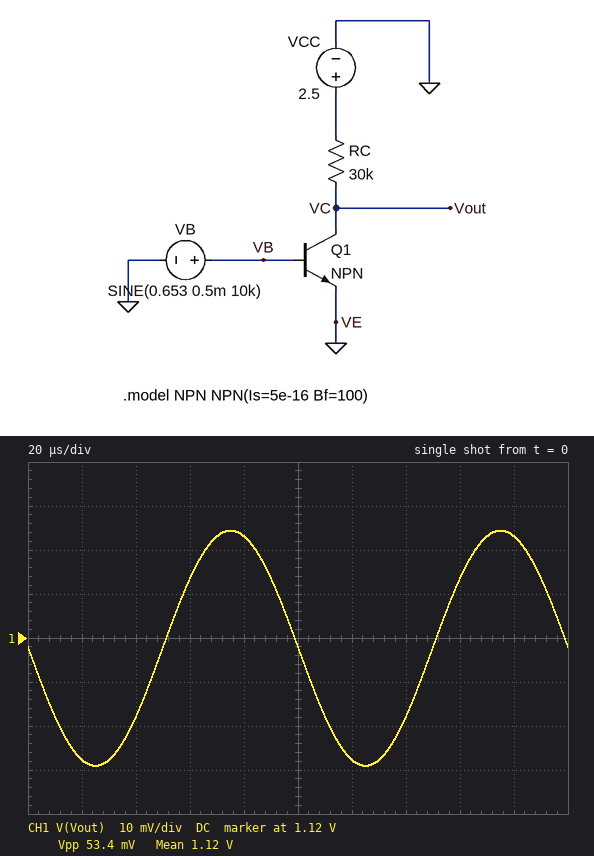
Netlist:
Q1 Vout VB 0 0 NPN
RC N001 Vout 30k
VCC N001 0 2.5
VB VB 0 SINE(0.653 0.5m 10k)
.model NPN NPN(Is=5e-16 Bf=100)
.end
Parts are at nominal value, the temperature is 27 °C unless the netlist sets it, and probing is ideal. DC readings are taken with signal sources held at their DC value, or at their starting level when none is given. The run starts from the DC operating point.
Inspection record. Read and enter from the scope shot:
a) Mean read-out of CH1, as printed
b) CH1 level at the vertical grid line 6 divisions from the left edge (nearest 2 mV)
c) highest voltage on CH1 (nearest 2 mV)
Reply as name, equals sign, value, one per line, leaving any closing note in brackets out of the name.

Mean read-out of CH1, as printed = 1.12 V
CH1 level at the vertical grid line 6 divisions from the left edge = 1.092 V
highest voltage on CH1 = 1.144 V
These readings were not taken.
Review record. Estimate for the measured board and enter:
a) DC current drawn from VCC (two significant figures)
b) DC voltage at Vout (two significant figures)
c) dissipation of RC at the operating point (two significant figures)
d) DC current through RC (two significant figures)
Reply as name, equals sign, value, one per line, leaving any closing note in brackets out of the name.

DC current drawn from VCC = 46 µA
DC voltage at Vout = 1.1 V
dissipation of RC at the operating point = 64 µW
DC current through RC = 46 µA
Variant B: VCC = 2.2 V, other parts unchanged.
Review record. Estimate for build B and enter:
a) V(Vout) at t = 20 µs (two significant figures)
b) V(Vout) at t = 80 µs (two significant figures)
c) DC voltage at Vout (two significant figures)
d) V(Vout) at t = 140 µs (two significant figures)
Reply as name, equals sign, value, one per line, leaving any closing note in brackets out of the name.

V(Vout) at t = 20 µs = 790 mV
V(Vout) at t = 80 µs = 840 mV
DC voltage at Vout = 820 mV
V(Vout) at t = 140 µs = 800 mV
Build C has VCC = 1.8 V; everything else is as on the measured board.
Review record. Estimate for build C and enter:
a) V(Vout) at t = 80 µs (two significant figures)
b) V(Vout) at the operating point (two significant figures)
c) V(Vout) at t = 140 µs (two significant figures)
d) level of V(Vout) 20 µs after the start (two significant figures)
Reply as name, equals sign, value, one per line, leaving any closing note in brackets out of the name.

V(Vout) at t = 80 µs = 440 mV
V(Vout) at the operating point = 420 mV
V(Vout) at t = 140 µs = 400 mV
level of V(Vout) 20 µs after the start = 390 mV
